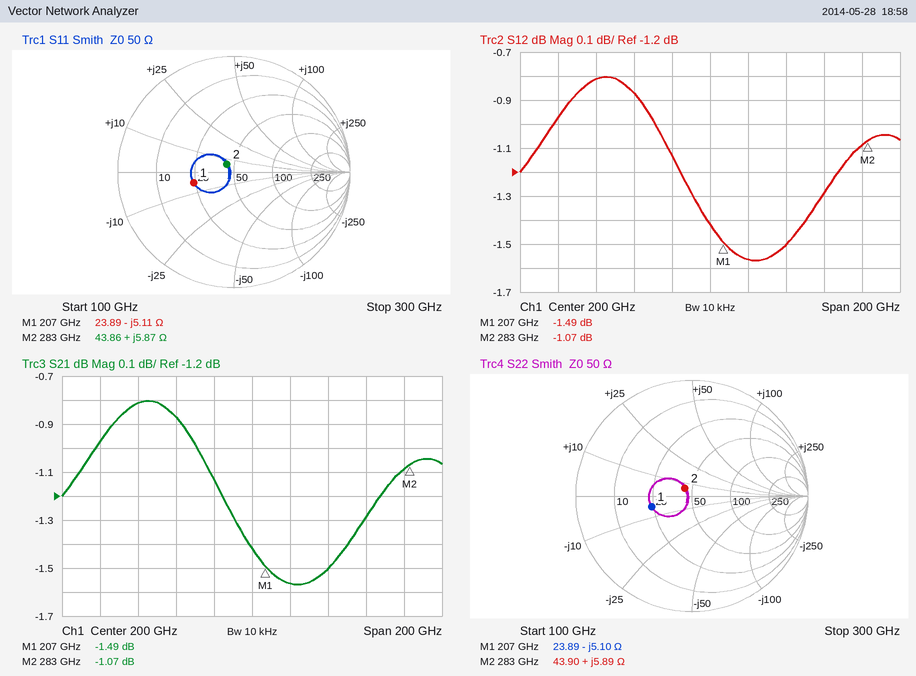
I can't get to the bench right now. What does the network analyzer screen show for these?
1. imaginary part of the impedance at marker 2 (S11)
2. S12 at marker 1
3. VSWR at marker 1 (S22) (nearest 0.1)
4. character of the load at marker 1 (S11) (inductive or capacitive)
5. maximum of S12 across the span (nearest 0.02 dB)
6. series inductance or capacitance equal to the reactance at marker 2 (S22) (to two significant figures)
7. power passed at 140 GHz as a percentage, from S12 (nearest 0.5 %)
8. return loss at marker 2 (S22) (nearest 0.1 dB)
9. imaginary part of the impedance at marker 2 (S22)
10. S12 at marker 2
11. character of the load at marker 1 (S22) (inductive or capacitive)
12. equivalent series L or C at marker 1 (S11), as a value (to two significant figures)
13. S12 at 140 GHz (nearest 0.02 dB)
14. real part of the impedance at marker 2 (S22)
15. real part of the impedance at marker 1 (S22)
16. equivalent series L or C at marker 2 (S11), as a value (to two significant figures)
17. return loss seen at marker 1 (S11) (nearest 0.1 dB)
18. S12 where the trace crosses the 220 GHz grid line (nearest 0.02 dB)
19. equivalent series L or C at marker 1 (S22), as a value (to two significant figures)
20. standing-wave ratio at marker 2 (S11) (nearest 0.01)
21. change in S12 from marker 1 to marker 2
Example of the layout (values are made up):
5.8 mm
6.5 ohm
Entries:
+5.87 Ω
-1.49 dB
2.1
capacitive
-0.80 dB
3.3 pH
83.0 %
20.9 dB
+5.89 Ω
-1.07 dB
capacitive
150 fF
-0.82 dB
43.90 Ω
23.89 Ω
3.3 pH
8.9 dB
-1.56 dB
150 fF
1.20
0.42 dB
